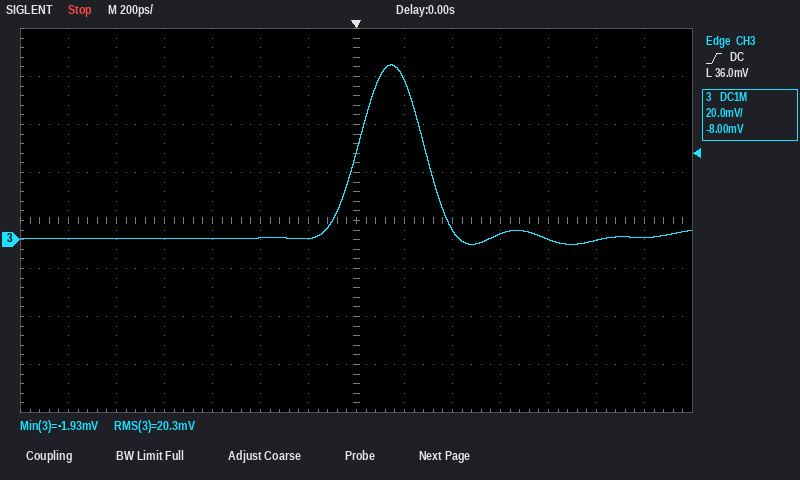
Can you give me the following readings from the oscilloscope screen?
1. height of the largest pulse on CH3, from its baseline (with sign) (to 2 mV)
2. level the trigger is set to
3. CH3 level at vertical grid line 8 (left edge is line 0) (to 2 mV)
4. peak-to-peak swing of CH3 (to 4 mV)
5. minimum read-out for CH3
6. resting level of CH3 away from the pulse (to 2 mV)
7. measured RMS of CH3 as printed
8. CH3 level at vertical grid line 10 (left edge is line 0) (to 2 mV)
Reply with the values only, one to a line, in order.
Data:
+72 mV
36.0 mV
66 mV
76 mV
-1.93 mV
0 mV
20.3 mV
2 mV
